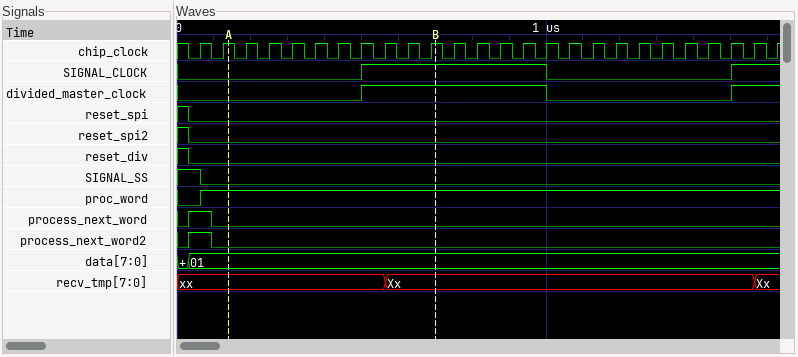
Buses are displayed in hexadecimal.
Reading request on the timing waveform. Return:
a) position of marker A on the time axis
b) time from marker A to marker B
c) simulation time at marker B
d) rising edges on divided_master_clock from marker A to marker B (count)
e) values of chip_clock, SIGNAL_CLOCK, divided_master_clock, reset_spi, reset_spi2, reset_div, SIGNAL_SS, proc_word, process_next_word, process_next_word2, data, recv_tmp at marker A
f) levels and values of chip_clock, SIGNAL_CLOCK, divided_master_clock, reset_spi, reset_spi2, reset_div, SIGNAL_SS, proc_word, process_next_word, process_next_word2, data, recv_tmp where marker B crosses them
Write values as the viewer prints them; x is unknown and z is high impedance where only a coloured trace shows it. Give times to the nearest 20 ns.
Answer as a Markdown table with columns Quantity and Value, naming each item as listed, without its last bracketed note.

| Quantity | Value |
|---|---|
| position of marker A on the time axis | 140 ns |
| time from marker A to marker B | 560 ns |
| simulation time at marker B | 700 ns |
| rising edges on divided_master_clock from marker A to marker B | 1 |
| values of chip_clock, SIGNAL_CLOCK, divided_master_clock, reset_spi, reset_spi2, reset_div, SIGNAL_SS, proc_word, process_next_word, process_next_word2, data, recv_tmp at marker A | chip_clock=1, SIGNAL_CLOCK=0, divided_master_clock=0, reset_spi=0, reset_spi2=0, reset_div=0, SIGNAL_SS=0, proc_word=1, process_next_word=0, process_next_word2=0, data=01, recv_tmp=xx |
| levels and values of chip_clock, SIGNAL_CLOCK, divided_master_clock, reset_spi, reset_spi2, reset_div, SIGNAL_SS, proc_word, process_next_word, process_next_word2, data, recv_tmp where marker B crosses them | chip_clock=1, SIGNAL_CLOCK=1, divided_master_clock=1, reset_spi=0, reset_spi2=0, reset_div=0, SIGNAL_SS=0, proc_word=1, process_next_word=0, process_next_word2=0, data=01, recv_tmp=Xx |
